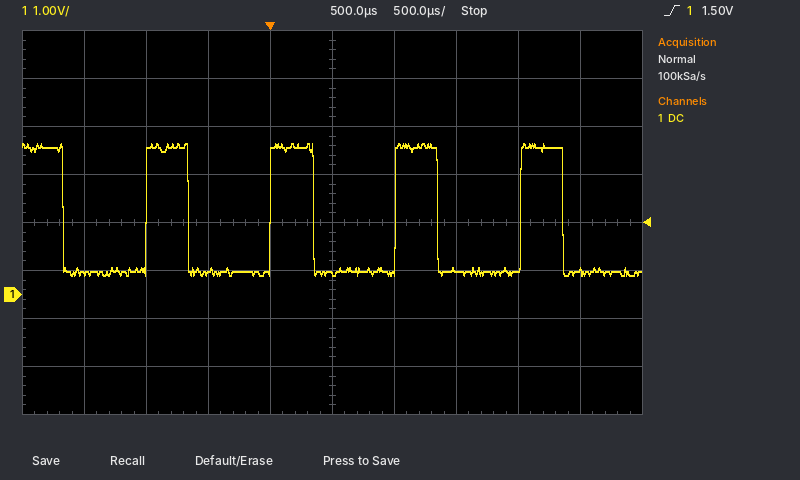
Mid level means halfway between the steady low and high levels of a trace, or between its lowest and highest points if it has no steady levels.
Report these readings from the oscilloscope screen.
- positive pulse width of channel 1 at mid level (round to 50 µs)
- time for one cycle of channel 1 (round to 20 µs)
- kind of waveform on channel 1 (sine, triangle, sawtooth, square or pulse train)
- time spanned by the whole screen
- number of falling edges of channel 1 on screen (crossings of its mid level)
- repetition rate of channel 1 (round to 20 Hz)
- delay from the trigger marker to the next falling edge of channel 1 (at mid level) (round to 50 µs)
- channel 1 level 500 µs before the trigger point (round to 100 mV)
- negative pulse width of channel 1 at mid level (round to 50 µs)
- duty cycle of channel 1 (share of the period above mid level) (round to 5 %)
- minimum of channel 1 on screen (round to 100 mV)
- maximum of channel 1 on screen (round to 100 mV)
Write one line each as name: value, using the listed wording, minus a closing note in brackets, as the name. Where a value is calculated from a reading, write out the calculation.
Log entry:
positive pulse width of channel 1 at mid level: 350 µs
time for one cycle of channel 1: 1.00 ms
kind of waveform on channel 1: pulse train
time spanned by the whole screen: 5 ms
number of falling edges of channel 1 on screen: 5
repetition rate of channel 1: 1 / 1.00 ms ≈ 1.00 kHz
delay from the trigger marker to the next falling edge of channel 1 (at mid level): 350 µs
channel 1 level 500 µs before the trigger point: 500 mV
negative pulse width of channel 1 at mid level: 650 µs
duty cycle of channel 1 (share of the period above mid level): 350 µs / 1.00 ms ≈ 35 %
minimum of channel 1 on screen: 400 mV
maximum of channel 1 on screen: 3.1 V
